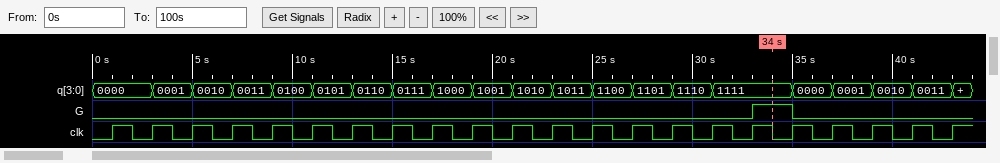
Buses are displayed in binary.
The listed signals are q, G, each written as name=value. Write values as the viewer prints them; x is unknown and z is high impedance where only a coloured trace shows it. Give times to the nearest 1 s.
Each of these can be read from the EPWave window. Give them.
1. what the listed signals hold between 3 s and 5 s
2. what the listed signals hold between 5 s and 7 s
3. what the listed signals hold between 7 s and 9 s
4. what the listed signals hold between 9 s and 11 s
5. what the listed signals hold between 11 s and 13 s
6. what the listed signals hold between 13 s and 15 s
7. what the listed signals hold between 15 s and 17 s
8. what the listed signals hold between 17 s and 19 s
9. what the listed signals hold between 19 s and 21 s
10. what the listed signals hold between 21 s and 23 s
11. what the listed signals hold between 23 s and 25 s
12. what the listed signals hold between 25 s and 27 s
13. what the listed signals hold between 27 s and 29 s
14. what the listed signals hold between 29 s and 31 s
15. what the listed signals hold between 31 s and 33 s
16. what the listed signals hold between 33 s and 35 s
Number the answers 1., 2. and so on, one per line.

1. q=0001, G=0
2. q=0010, G=0
3. q=0011, G=0
4. q=0100, G=0
5. q=0101, G=0
6. q=0110, G=0
7. q=0111, G=0
8. q=1000, G=0
9. q=1001, G=0
10. q=1010, G=0
11. q=1011, G=0
12. q=1100, G=0
13. q=1101, G=0
14. q=1110, G=0
15. q=1111, G=0
16. q=1111, G=1
